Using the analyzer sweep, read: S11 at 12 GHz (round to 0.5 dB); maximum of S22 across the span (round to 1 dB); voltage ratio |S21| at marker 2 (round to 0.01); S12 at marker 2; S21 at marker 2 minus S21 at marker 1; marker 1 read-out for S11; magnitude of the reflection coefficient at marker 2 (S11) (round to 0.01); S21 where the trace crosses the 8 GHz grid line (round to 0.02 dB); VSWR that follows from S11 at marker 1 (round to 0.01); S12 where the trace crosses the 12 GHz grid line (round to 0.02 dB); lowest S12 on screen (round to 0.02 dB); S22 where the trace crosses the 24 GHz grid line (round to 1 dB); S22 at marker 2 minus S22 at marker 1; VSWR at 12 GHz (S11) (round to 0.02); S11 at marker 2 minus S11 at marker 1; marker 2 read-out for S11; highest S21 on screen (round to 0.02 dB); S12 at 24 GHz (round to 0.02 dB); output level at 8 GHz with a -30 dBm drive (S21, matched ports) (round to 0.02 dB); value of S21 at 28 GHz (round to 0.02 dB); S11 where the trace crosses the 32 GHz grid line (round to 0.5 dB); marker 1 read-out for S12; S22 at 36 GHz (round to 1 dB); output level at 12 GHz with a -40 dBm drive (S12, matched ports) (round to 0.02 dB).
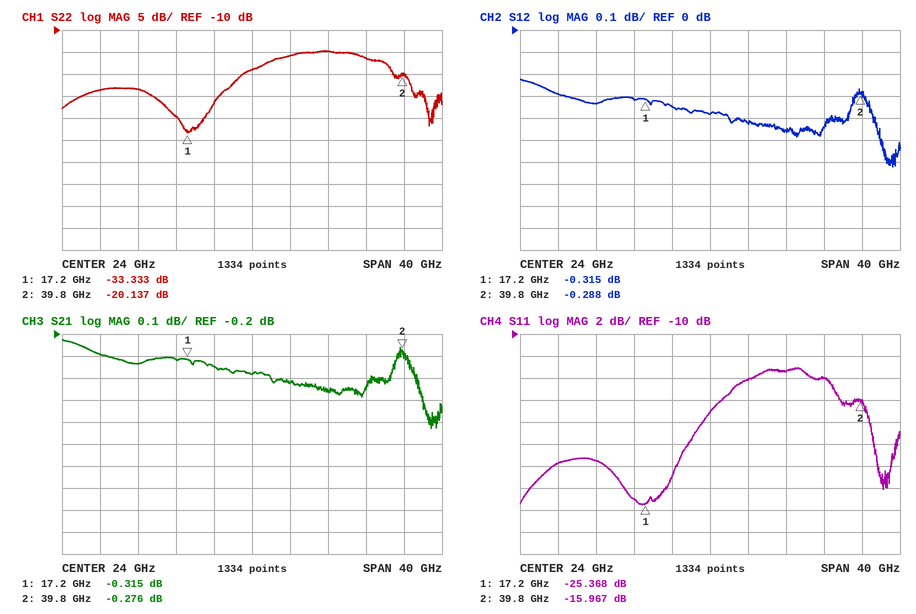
-21.5 dB
-15 dB
0.97
-0.288 dB
0.039 dB
-25.368 dB
0.16
-0.30 dB
1.11
-0.34 dB
-0.62 dB
-19 dB
13.196 dB
1.18
9.401 dB
-15.967 dB
-0.22 dB
-0.38 dB
-30.30 dBm
-0.42 dB
-13.5 dB
-0.315 dB
-16 dB
-40.34 dBm
